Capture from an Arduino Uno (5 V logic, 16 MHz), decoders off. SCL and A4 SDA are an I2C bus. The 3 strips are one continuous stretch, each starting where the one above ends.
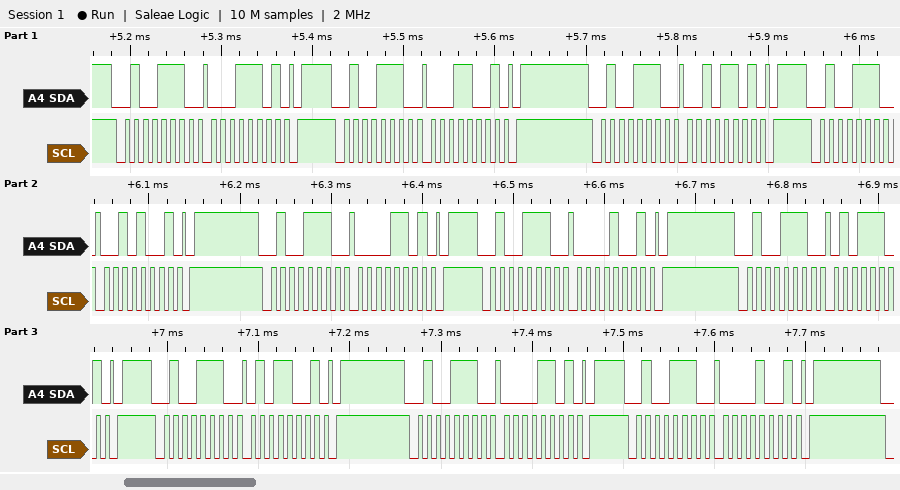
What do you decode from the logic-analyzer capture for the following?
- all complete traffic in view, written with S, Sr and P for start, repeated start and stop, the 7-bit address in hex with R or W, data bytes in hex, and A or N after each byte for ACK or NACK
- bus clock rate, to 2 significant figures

S 27W A 1D A P S 27W A 19 A P S 27W A 2D A P S 27W A 29 A P S 27W A 0D A P S 27W A 09 A P S 27W A 5D A P S 27W A 59 A P S 27W A 0D A P S 27W A 09 A P
100 kHz
